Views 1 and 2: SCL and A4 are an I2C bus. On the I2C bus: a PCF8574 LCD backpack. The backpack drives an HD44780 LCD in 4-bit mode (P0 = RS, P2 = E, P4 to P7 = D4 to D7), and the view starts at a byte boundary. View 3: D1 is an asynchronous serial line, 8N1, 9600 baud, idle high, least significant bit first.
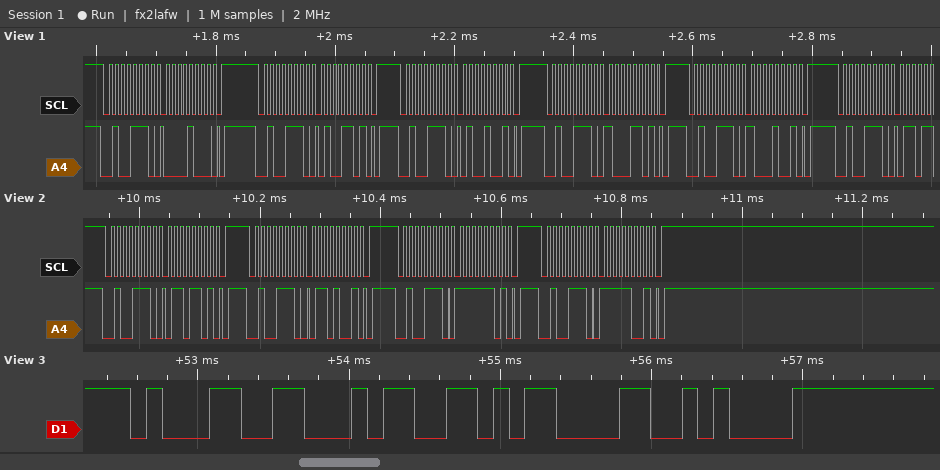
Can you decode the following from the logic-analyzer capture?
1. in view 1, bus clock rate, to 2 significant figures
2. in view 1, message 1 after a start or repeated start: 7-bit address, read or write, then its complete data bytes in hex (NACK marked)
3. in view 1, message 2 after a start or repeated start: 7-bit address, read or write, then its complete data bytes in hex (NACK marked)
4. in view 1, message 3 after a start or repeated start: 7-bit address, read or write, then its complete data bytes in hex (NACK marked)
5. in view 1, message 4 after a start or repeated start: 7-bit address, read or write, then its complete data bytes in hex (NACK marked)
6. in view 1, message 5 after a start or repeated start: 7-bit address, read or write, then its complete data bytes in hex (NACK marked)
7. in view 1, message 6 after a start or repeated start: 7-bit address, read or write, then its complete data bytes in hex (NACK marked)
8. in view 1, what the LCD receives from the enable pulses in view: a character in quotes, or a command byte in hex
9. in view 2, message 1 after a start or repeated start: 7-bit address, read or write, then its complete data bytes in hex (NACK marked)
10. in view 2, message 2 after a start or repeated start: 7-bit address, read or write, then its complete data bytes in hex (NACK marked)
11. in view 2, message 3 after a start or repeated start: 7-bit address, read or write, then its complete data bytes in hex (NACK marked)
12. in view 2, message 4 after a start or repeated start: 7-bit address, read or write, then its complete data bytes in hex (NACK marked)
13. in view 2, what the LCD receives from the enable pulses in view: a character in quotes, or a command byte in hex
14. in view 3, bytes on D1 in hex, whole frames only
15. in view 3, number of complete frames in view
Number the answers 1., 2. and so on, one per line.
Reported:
1. 100 kHz
2. 0x27 write: 08
3. 0x27 write: 4D
4. 0x27 write: 49
5. 0x27 write: 8D
6. 0x27 write: 89
7. 0x27 write
8. 'H'
9. 0x27 write: 6D
10. 0x27 write: 69
11. 0x27 write: FD
12. 0x27 write: F9
13. 'o'
14. 0x31 0x34 0x0D 0x0A
15. 4
